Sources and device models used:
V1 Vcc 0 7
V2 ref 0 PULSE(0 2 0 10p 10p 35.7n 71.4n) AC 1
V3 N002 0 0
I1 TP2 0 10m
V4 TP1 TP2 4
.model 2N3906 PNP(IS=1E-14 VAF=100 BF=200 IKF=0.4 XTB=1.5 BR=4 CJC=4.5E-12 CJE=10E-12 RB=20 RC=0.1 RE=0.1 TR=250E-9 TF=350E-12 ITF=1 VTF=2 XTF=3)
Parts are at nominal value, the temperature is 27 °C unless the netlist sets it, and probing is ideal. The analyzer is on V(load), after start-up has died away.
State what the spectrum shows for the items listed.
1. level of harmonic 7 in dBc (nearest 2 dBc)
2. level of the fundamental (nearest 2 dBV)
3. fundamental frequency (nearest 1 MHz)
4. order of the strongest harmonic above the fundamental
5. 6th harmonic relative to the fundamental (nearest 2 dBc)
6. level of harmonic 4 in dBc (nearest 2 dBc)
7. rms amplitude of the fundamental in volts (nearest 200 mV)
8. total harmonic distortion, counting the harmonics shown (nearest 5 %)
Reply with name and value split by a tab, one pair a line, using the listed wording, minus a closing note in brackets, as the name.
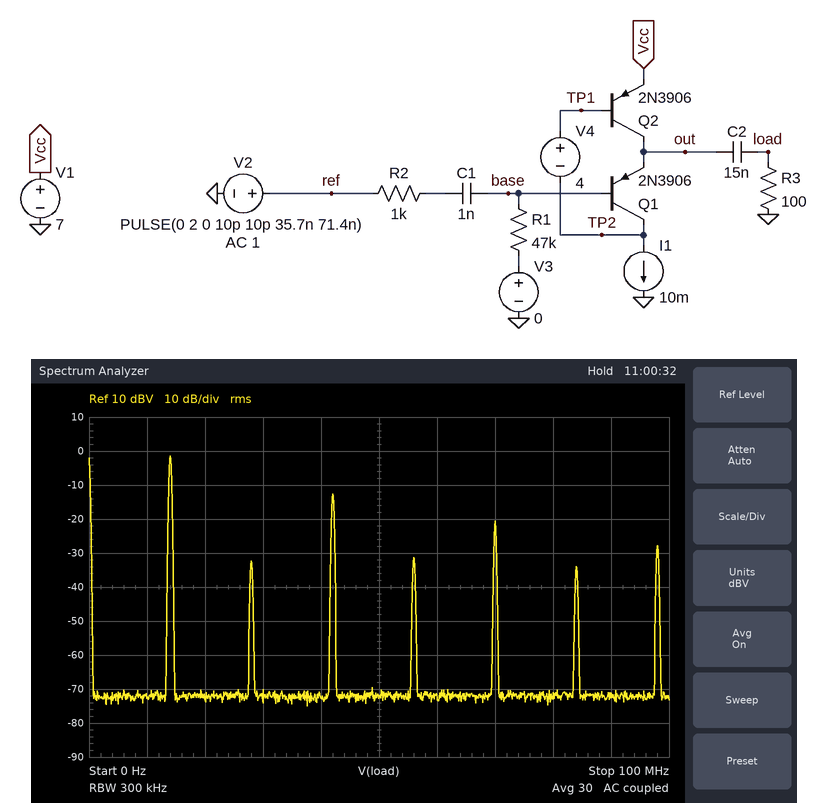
level of harmonic 7 in dBc	-26 dBc
level of the fundamental	-2 dBV
fundamental frequency	14 MHz
order of the strongest harmonic above the fundamental	3
6th harmonic relative to the fundamental	-32 dBc
level of harmonic 4 in dBc	-30 dBc
rms amplitude of the fundamental in volts	800 mV
total harmonic distortion, counting the harmonics shown	30 %
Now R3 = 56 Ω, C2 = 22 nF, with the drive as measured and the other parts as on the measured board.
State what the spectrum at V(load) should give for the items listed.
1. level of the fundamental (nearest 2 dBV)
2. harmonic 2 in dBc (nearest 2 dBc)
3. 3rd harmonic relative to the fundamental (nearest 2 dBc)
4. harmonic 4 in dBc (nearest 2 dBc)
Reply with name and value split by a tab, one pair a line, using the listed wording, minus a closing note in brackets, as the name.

level of the fundamental	-4 dBV
harmonic 2 in dBc	-8 dBc
3rd harmonic relative to the fundamental	-24 dBc
harmonic 4 in dBc	-14 dBc
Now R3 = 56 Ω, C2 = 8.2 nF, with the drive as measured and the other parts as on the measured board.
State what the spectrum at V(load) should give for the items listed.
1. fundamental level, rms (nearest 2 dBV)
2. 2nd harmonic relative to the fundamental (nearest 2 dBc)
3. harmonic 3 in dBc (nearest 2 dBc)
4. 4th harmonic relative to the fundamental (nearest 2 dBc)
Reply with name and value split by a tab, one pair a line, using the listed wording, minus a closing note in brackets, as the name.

fundamental level, rms	-4 dBV
2nd harmonic relative to the fundamental	-8 dBc
harmonic 3 in dBc	-22 dBc
4th harmonic relative to the fundamental	-14 dBc
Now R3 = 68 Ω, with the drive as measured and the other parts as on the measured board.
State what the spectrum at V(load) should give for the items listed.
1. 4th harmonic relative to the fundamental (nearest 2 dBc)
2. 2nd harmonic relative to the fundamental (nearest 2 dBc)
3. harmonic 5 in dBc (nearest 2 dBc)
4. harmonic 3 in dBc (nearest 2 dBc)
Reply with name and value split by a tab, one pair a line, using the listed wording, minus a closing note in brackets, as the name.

4th harmonic relative to the fundamental	-14 dBc
2nd harmonic relative to the fundamental	-12 dBc
harmonic 5 in dBc	-34 dBc
harmonic 3 in dBc	-14 dBc
